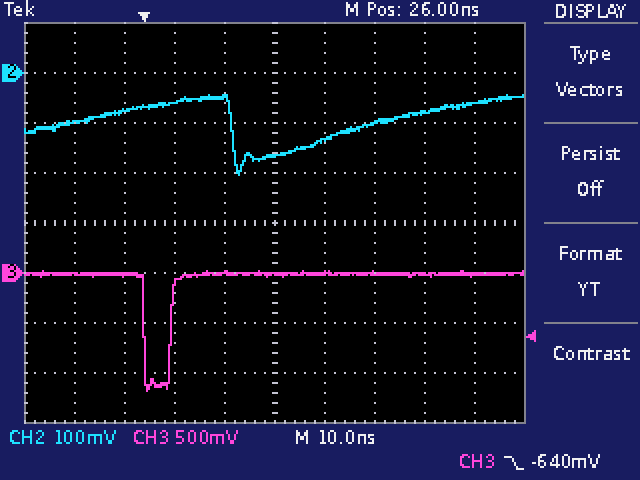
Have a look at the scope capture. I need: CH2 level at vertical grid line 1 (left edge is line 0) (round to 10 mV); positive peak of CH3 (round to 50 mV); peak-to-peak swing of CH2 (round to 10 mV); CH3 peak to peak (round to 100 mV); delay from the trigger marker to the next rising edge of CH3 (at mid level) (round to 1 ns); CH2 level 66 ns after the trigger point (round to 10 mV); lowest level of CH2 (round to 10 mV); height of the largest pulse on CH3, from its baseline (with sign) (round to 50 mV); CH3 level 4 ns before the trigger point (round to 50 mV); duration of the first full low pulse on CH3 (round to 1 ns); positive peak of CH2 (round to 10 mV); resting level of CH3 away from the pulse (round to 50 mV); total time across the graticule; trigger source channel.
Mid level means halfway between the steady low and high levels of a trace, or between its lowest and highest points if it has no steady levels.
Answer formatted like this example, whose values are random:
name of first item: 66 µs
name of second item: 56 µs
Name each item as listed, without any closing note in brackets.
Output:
CH2 level at vertical grid line 1 (left edge is line 0): -100 mV
positive peak of CH3: 0 mV
peak-to-peak swing of CH2: 160 mV
CH3 peak to peak: 1.20 V
delay from the trigger marker to the next rising edge of CH3 (at mid level): 5 ns
CH2 level 66 ns after the trigger point: -60 mV
lowest level of CH2: -200 mV
height of the largest pulse on CH3, from its baseline (with sign): -1.15 V
CH3 level 4 ns before the trigger point: 0 mV
duration of the first full low pulse on CH3: 5 ns
positive peak of CH2: -40 mV
resting level of CH3 away from the pulse: 0 mV
total time across the graticule: 100 ns
trigger source channel: CH3
